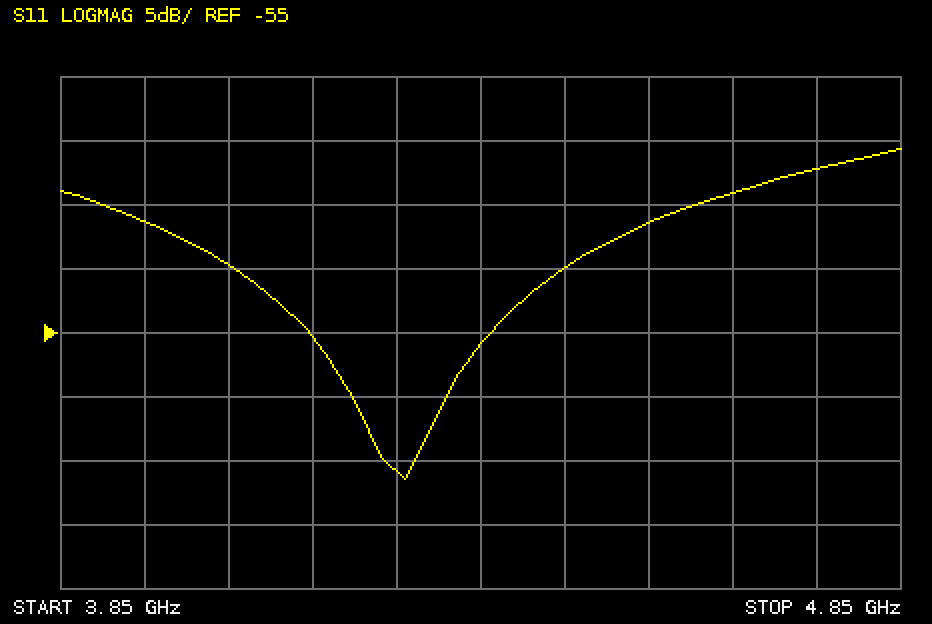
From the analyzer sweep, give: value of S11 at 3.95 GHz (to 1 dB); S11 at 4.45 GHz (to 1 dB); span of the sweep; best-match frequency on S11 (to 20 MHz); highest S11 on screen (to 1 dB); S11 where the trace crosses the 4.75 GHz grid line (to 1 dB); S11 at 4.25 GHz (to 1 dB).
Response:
-46 dB
-50 dB
1 GHz
4.26 GHz
-41 dB
-42 dB
-66 dB
